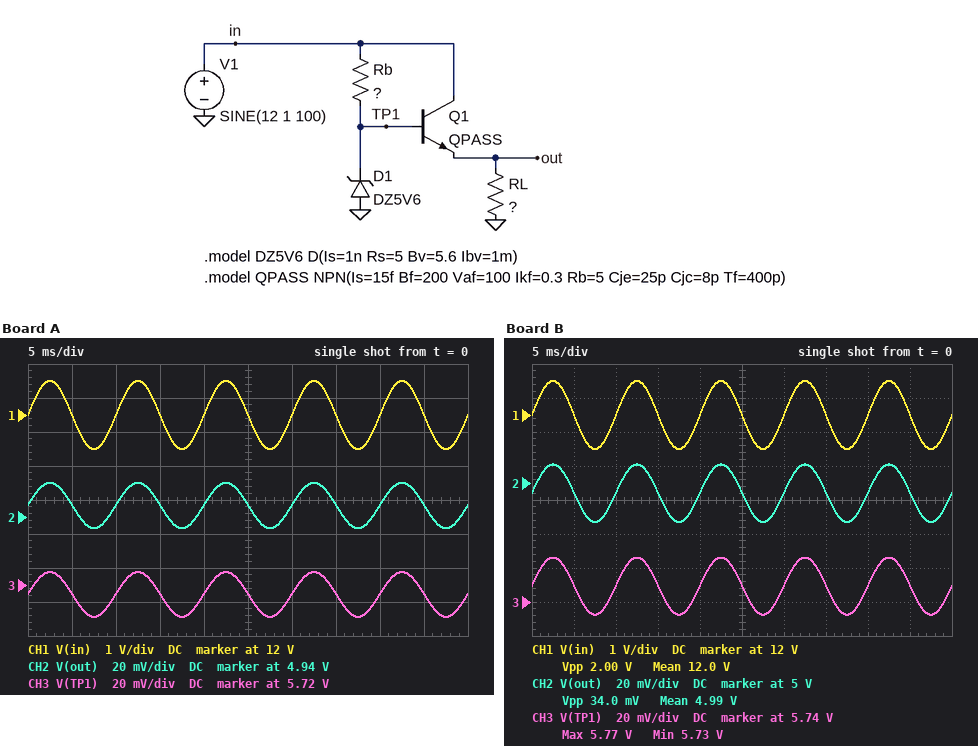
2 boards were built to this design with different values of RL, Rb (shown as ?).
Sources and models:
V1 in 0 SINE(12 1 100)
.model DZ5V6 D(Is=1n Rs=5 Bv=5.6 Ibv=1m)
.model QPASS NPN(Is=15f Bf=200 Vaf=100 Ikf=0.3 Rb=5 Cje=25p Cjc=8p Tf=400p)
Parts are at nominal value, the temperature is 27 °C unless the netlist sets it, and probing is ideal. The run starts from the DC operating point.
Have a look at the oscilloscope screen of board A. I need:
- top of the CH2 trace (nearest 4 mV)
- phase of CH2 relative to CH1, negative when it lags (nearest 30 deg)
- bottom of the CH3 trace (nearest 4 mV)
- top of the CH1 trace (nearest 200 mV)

4.960 V
0 deg
5.700 V
13.0 V
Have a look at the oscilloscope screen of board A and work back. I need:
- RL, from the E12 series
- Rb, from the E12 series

56 Ω
560 Ω
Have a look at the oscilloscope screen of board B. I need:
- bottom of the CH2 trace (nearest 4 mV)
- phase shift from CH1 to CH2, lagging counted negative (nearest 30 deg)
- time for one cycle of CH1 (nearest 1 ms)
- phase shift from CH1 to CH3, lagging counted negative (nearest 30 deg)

4.976 V
0 deg
10 ms
0 deg
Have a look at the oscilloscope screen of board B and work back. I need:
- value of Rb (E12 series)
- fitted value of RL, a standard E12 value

390 Ω
82 Ω
